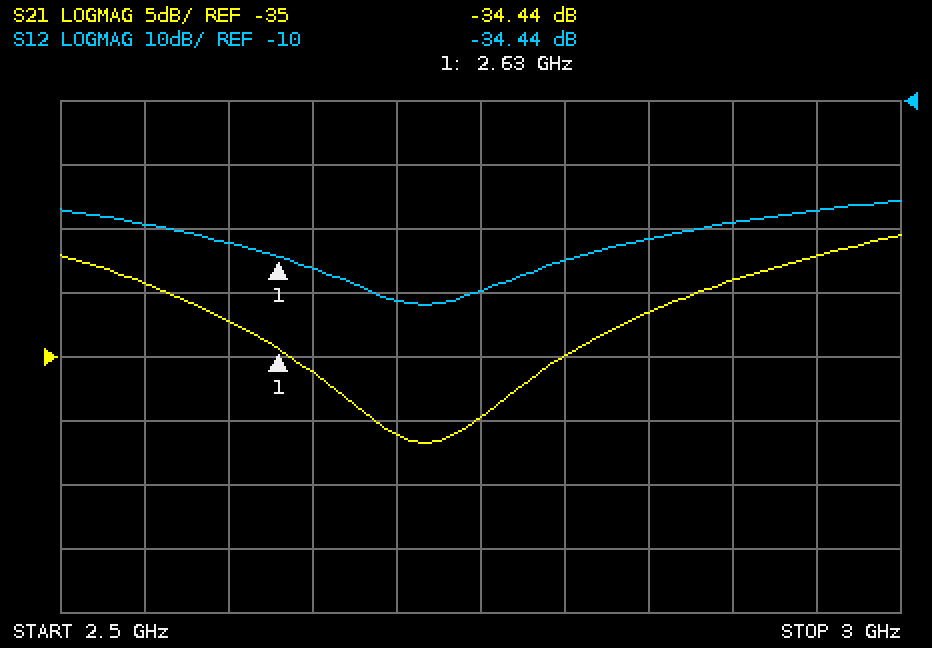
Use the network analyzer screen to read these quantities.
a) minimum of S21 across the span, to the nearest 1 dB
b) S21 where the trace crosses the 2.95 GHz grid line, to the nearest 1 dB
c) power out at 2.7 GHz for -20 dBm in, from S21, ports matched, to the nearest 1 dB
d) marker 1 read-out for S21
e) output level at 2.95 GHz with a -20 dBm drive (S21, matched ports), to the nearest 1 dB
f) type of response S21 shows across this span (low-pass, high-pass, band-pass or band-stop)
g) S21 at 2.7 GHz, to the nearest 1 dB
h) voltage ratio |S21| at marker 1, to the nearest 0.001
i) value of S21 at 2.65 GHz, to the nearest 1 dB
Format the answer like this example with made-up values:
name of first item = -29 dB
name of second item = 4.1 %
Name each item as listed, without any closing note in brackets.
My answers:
minimum of S21 across the span, to the nearest 1 dB = -42 dB
S21 where the trace crosses the 2.95 GHz grid line, to the nearest 1 dB = -27 dB
power out at 2.7 GHz for -20 dBm in, from S21, ports matched, to the nearest 1 dB = -61 dBm
marker 1 read-out for S21 = -34.44 dB
output level at 2.95 GHz with a -20 dBm drive (S21, matched ports), to the nearest 1 dB = -47 dBm
type of response S21 shows across this span = band-stop
S21 at 2.7 GHz, to the nearest 1 dB = -41 dB
voltage ratio |S21| at marker 1, to the nearest 0.001 = 0.019
value of S21 at 2.65 GHz, to the nearest 1 dB = -36 dB
